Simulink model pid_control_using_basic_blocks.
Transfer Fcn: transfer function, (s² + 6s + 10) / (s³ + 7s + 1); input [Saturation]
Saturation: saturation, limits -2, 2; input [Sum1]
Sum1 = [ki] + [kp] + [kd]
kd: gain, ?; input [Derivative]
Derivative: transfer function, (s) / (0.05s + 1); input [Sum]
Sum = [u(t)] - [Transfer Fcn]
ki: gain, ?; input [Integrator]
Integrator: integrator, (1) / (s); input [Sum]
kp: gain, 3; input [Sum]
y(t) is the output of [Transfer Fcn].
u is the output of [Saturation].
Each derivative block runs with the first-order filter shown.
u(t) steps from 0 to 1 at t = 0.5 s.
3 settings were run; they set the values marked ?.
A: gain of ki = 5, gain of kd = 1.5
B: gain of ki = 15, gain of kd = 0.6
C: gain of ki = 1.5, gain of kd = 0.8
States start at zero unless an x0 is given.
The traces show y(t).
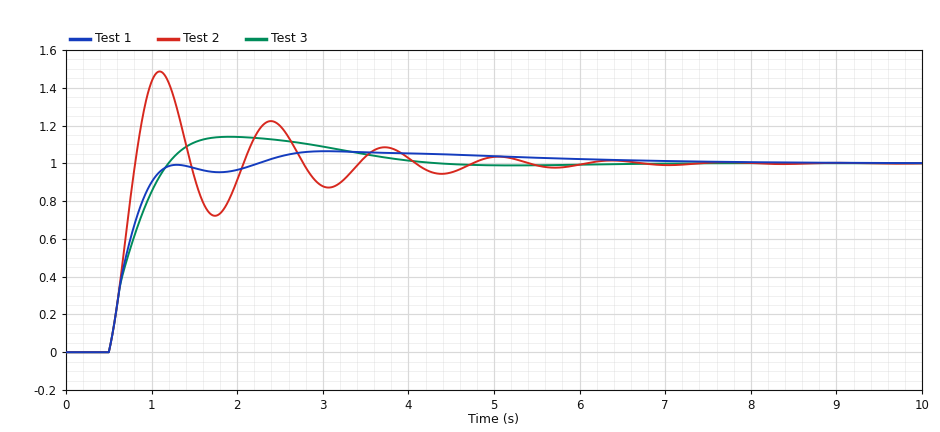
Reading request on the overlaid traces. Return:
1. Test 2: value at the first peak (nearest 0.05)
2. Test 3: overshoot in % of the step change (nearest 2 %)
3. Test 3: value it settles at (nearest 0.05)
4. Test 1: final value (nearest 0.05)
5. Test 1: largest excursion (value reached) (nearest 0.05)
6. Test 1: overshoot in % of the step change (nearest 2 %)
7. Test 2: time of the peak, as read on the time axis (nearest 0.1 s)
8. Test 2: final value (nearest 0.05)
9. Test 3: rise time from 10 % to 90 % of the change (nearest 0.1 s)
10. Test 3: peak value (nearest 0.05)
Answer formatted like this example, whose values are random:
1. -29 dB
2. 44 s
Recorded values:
1. 1.50
2. 14 %
3. 1.00
4. 1.00
5. 1.05
6. 6 %
7. 1.1 s
8. 1.00
9. 0.5 s
10. 1.15
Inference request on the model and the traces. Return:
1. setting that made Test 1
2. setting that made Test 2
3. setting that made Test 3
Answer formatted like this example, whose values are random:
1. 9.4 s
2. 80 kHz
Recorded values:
1. C
2. B
3. A
